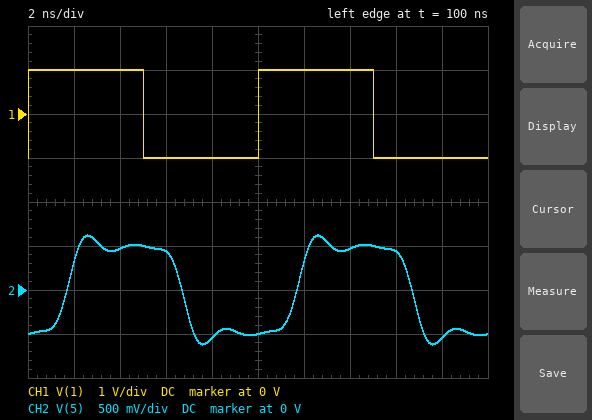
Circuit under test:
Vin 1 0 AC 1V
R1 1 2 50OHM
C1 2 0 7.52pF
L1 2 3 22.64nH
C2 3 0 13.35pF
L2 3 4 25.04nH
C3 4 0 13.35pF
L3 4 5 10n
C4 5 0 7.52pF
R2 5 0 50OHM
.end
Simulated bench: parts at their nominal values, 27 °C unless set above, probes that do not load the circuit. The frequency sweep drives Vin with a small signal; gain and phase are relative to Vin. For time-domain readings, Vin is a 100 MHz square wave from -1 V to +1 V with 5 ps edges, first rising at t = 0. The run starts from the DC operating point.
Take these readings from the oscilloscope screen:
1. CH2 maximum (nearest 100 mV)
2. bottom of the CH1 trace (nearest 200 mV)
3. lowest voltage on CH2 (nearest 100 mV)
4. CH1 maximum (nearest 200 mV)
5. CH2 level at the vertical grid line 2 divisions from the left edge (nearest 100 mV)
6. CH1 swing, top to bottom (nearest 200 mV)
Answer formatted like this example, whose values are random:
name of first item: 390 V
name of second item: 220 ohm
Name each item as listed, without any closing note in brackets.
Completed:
CH2 maximum: 600 mV
bottom of the CH1 trace: -1.0 V
lowest voltage on CH2: -600 mV
CH1 maximum: 1.0 V
CH2 level at the vertical grid line 2 divisions from the left edge: 500 mV
CH1 swing, top to bottom: 2.0 V
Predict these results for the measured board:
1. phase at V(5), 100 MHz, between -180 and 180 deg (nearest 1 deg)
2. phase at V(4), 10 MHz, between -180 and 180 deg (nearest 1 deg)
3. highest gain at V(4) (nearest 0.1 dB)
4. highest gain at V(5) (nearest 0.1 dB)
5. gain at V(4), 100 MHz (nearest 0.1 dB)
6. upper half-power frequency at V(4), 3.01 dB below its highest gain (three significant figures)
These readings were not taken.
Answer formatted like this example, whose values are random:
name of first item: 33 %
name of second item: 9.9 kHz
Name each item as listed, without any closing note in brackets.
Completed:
phase at V(5), 100 MHz, between -180 and 180 deg: -57 deg
phase at V(4), 10 MHz, between -180 and 180 deg: -5 deg
highest gain at V(4): -6.0 dB
highest gain at V(5): -6.0 dB
gain at V(4), 100 MHz: -6.4 dB
upper half-power frequency at V(4), 3.01 dB below its highest gain: 328 MHz
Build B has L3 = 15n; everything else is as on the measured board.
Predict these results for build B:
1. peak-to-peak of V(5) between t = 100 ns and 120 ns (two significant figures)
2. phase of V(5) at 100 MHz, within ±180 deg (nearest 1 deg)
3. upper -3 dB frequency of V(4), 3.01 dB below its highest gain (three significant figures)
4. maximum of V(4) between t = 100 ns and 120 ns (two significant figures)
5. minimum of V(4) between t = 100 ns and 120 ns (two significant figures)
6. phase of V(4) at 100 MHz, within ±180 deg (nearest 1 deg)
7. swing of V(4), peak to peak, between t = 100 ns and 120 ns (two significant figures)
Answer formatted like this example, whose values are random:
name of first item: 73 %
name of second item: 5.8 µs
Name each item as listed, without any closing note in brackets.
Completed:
peak-to-peak of V(5) between t = 100 ns and 120 ns: 1.3 V
phase of V(5) at 100 MHz, within ±180 deg: -59 deg
upper -3 dB frequency of V(4), 3.01 dB below its highest gain: 542 MHz
maximum of V(4) between t = 100 ns and 120 ns: 540 mV
minimum of V(4) between t = 100 ns and 120 ns: -540 mV
phase of V(4) at 100 MHz, within ±180 deg: -48 deg
swing of V(4), peak to peak, between t = 100 ns and 120 ns: 1.1 V
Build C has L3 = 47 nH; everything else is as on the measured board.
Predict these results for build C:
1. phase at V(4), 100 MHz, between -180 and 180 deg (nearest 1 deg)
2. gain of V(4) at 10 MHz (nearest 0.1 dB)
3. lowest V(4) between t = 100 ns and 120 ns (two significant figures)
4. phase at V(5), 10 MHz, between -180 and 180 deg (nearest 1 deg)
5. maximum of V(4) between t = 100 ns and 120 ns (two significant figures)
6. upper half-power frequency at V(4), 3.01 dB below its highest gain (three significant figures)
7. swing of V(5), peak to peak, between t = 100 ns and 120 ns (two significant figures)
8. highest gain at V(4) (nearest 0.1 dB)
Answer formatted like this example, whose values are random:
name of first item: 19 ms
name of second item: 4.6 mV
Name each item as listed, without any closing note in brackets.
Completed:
phase at V(4), 100 MHz, between -180 and 180 deg: -38 deg
gain of V(4) at 10 MHz: -6.0 dB
lowest V(4) between t = 100 ns and 120 ns: -970 mV
phase at V(5), 10 MHz, between -180 and 180 deg: -7 deg
maximum of V(4) between t = 100 ns and 120 ns: 970 mV
upper half-power frequency at V(4), 3.01 dB below its highest gain: 511 MHz
swing of V(5), peak to peak, between t = 100 ns and 120 ns: 1.3 V
highest gain at V(4): -0.3 dB
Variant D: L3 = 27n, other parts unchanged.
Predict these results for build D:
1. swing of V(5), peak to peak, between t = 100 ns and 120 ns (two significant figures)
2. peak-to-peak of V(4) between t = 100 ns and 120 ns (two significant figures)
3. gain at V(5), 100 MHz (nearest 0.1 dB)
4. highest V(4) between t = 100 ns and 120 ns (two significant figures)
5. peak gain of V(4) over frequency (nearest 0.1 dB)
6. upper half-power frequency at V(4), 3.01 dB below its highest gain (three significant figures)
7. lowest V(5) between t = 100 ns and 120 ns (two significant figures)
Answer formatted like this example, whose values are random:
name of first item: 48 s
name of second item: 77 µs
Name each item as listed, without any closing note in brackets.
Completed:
swing of V(5), peak to peak, between t = 100 ns and 120 ns: 1.4 V
peak-to-peak of V(4) between t = 100 ns and 120 ns: 1.6 V
gain at V(5), 100 MHz: -6.1 dB
highest V(4) between t = 100 ns and 120 ns: 780 mV
peak gain of V(4) over frequency: -0.8 dB
upper half-power frequency at V(4), 3.01 dB below its highest gain: 529 MHz
lowest V(5) between t = 100 ns and 120 ns: -710 mV
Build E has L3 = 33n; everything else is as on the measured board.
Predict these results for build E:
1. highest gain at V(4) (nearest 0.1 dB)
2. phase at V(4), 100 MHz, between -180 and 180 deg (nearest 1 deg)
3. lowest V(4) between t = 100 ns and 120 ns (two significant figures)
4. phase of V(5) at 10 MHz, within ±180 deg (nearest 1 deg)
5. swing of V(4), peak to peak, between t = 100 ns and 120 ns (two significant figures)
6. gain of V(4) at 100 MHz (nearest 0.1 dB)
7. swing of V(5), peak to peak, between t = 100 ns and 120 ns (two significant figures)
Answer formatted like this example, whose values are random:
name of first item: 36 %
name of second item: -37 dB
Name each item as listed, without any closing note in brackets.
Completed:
highest gain at V(4): -0.2 dB
phase at V(4), 100 MHz, between -180 and 180 deg: -42 deg
lowest V(4) between t = 100 ns and 120 ns: -860 mV
phase of V(5) at 10 MHz, within ±180 deg: -7 deg
swing of V(4), peak to peak, between t = 100 ns and 120 ns: 1.7 V
gain of V(4) at 100 MHz: -6.1 dB
swing of V(5), peak to peak, between t = 100 ns and 120 ns: 1.4 V
